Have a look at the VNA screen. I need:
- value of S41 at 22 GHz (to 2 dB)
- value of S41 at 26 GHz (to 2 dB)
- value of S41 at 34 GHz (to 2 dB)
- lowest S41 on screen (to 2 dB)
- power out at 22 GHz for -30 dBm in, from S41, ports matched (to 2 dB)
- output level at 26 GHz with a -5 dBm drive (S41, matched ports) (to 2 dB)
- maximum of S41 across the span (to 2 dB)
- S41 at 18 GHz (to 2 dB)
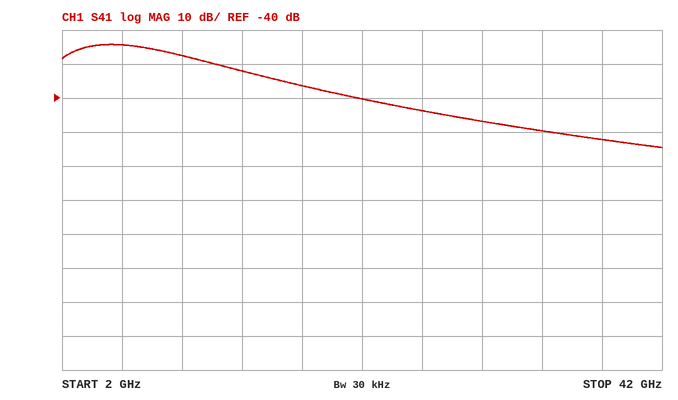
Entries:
-40 dB
-44 dB
-50 dB
-54 dB
-70 dBm
-48 dBm
-24 dB
-36 dB
